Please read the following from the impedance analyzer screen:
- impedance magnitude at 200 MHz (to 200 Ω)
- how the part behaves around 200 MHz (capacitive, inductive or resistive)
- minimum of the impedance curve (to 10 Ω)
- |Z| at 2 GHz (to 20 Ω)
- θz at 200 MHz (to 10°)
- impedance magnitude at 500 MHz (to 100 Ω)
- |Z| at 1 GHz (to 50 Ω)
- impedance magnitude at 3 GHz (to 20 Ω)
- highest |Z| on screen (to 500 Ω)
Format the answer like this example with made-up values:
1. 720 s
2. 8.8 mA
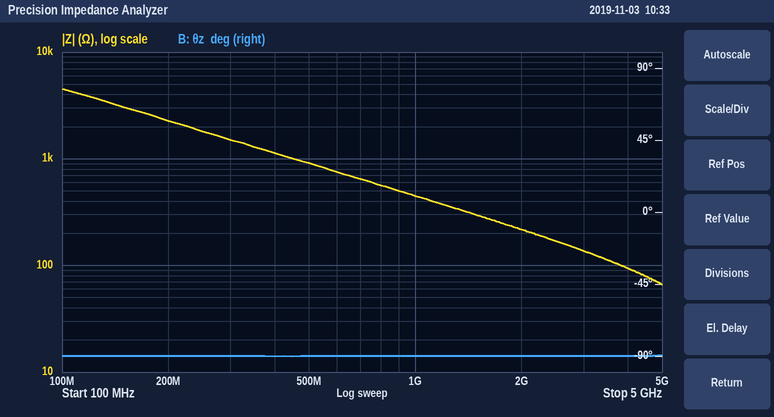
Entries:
1. 2.2 kΩ
2. capacitive
3. 70 Ω
4. 220 Ω
5. -90°
6. 900 Ω
7. 450 Ω
8. 140 Ω
9. 4.5 kΩ
